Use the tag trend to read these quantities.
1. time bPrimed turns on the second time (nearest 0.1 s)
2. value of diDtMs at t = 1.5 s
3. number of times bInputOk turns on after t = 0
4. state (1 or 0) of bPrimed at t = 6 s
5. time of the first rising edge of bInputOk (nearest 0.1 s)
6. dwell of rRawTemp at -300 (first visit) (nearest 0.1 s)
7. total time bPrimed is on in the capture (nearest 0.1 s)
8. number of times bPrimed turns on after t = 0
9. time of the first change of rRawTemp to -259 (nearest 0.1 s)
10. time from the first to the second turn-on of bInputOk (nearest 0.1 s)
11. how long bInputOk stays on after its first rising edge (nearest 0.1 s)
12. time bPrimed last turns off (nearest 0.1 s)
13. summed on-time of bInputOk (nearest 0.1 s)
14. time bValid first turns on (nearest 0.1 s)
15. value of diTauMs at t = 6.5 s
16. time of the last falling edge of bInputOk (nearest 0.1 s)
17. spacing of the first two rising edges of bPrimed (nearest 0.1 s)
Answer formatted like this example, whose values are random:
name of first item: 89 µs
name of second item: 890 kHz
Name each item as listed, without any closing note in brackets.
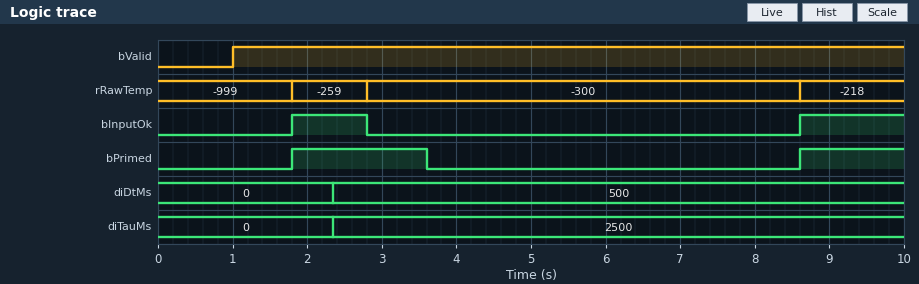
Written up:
time bPrimed turns on the second time: 8.6 s
value of diDtMs at t = 1.5 s: 0
number of times bInputOk turns on after t = 0: 2
state (1 or 0) of bPrimed at t = 6 s: 0
time of the first rising edge of bInputOk: 1.8 s
dwell of rRawTemp at -300 (first visit): 5.8 s
total time bPrimed is on in the capture: 3.2 s
number of times bPrimed turns on after t = 0: 2
time of the first change of rRawTemp to -259: 1.8 s
time from the first to the second turn-on of bInputOk: 6.8 s
how long bInputOk stays on after its first rising edge: 1.0 s
time bPrimed last turns off: 3.6 s
summed on-time of bInputOk: 2.4 s
time bValid first turns on: 1.0 s
value of diTauMs at t = 6.5 s: 2500
time of the last falling edge of bInputOk: 2.8 s
spacing of the first two rising edges of bPrimed: 6.8 s
